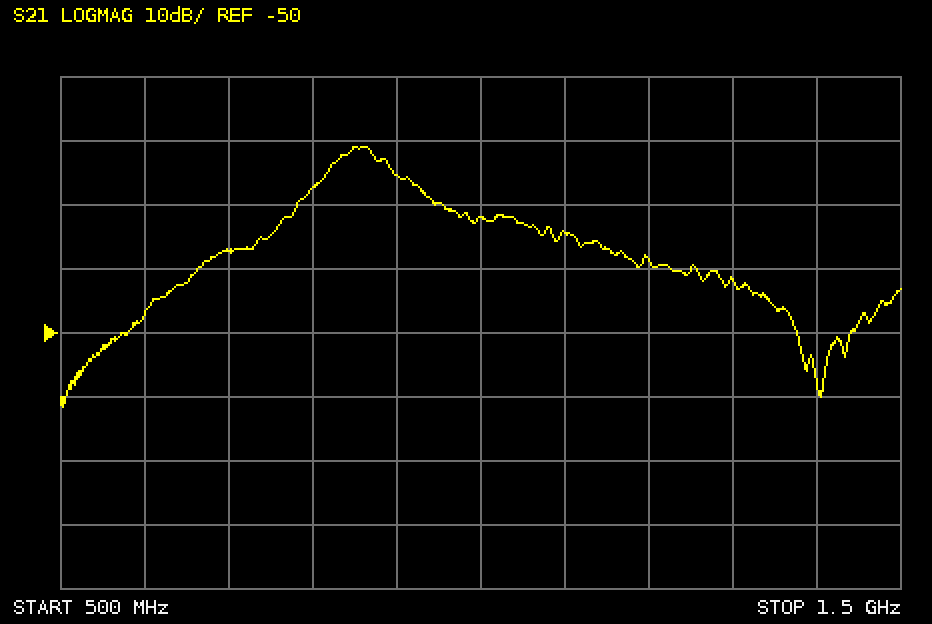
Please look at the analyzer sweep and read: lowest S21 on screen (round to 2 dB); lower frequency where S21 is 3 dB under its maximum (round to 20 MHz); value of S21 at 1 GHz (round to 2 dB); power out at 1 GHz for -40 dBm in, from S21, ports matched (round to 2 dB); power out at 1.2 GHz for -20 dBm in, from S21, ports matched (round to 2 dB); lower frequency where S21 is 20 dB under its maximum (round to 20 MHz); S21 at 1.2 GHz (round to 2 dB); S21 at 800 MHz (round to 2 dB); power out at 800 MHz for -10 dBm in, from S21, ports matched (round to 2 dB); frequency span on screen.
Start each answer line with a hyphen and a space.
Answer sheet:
- -62 dB
- 820 MHz
- -32 dB
- -72 dBm
- -58 dBm
- 660 MHz
- -38 dB
- -28 dB
- -38 dBm
- 1 GHz
